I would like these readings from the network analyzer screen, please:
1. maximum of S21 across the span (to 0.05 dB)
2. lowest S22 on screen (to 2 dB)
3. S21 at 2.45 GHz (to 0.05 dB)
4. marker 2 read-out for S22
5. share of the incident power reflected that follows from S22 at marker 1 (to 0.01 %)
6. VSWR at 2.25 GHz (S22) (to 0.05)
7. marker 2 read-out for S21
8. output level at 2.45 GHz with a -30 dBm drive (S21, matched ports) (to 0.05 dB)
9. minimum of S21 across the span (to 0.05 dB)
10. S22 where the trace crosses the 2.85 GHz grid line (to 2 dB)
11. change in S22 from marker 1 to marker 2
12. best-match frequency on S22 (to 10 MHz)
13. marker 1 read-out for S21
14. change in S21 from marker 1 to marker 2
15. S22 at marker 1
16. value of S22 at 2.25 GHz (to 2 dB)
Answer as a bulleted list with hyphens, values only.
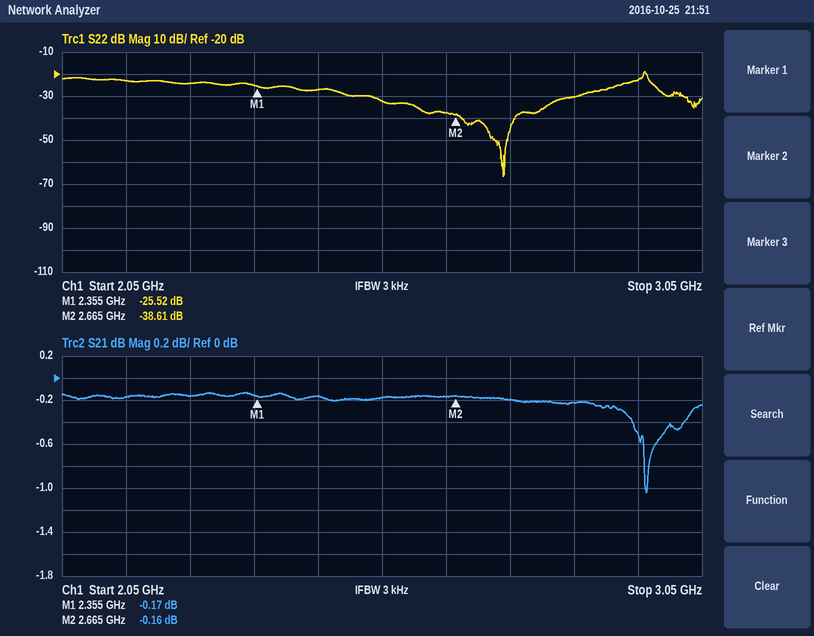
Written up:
- -0.15 dB
- -66 dB
- -0.15 dB
- -38.61 dB
- 0.28 %
- 1.15
- -0.16 dB
- -30.15 dBm
- -1.05 dB
- -30 dB
- -13.09 dB
- 2.74 GHz
- -0.17 dB
- 0.01 dB
- -25.52 dB
- -24 dB
